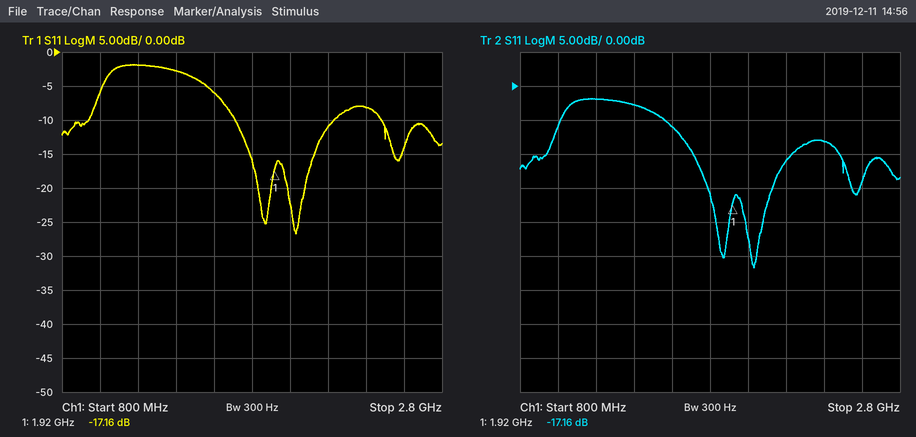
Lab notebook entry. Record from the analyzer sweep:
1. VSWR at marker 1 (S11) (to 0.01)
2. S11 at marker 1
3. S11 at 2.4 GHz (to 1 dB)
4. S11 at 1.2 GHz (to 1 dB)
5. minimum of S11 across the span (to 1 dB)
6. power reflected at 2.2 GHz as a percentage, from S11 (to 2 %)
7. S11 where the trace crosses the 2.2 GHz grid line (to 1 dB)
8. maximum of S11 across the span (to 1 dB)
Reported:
1.32
-17.16 dB
-8 dB
-2 dB
-27 dB
8 %
-11 dB
-2 dB
